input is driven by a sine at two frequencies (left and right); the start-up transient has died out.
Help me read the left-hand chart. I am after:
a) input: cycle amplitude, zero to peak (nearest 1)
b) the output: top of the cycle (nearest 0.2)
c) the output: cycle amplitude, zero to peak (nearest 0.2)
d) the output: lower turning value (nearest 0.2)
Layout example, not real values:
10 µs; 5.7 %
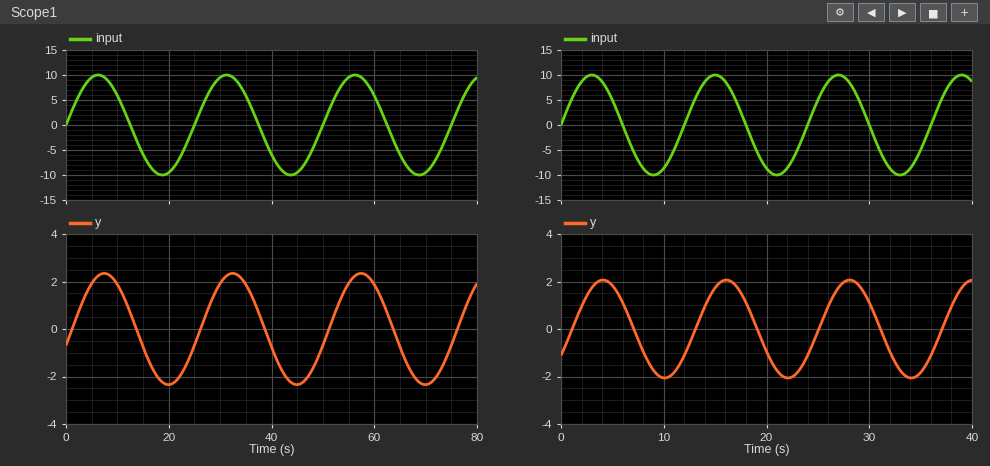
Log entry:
10; 2.4; 2.4; -2.4
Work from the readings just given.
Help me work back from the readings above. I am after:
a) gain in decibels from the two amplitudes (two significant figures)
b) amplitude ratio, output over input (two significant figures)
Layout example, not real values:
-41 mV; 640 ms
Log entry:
-12 dB; 0.24
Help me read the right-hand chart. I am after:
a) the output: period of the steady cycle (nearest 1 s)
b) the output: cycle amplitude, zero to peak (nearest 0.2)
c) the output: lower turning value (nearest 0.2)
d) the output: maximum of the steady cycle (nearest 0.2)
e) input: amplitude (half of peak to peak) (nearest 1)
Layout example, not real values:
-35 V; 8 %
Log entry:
12 s; 2.0; -2.0; 2.0; 10
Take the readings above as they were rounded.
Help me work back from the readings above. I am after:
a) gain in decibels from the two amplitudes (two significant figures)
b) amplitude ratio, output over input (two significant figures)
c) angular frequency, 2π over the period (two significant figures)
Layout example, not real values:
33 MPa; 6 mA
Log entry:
-14 dB; 0.20; 0.52 rad/s
